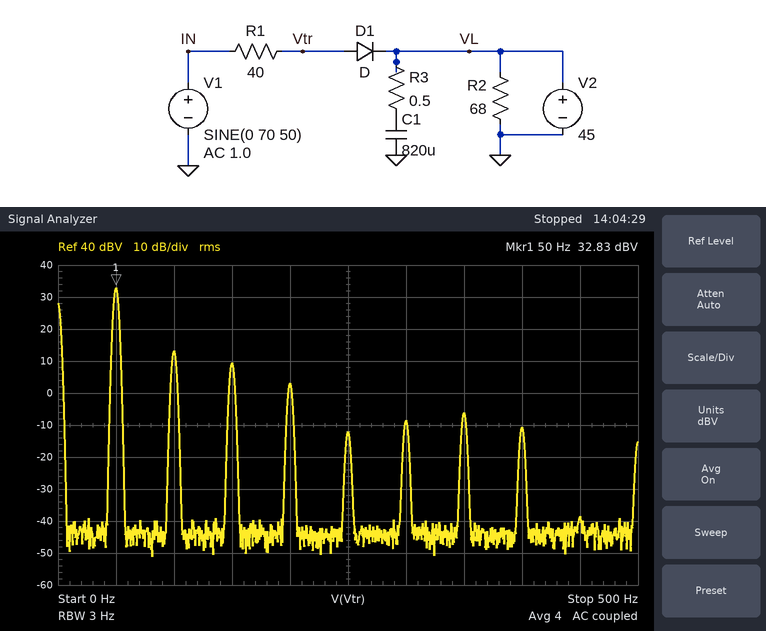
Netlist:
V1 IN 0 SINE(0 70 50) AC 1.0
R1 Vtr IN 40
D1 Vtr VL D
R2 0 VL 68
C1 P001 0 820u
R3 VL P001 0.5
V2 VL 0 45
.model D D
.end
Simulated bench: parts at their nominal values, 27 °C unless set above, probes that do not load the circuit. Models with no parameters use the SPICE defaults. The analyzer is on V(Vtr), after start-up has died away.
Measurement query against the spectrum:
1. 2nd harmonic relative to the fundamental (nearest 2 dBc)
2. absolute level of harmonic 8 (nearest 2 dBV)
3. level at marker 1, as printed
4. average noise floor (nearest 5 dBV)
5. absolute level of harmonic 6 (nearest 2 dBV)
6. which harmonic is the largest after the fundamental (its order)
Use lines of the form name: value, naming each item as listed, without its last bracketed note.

2nd harmonic relative to the fundamental: -20 dBc
absolute level of harmonic 8: -10 dBV
level at marker 1, as printed: 32.83 dBV
average noise floor: -45 dBV
absolute level of harmonic 6: -8 dBV
which harmonic is the largest after the fundamental: 2
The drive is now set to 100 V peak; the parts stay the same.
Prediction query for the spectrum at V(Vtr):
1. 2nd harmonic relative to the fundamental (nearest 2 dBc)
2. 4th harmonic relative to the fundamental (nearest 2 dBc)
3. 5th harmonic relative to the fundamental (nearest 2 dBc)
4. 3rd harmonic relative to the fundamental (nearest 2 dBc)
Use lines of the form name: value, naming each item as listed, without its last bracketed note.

2nd harmonic relative to the fundamental: -14 dBc
4th harmonic relative to the fundamental: -40 dBc
5th harmonic relative to the fundamental: -32 dBc
3rd harmonic relative to the fundamental: -22 dBc
